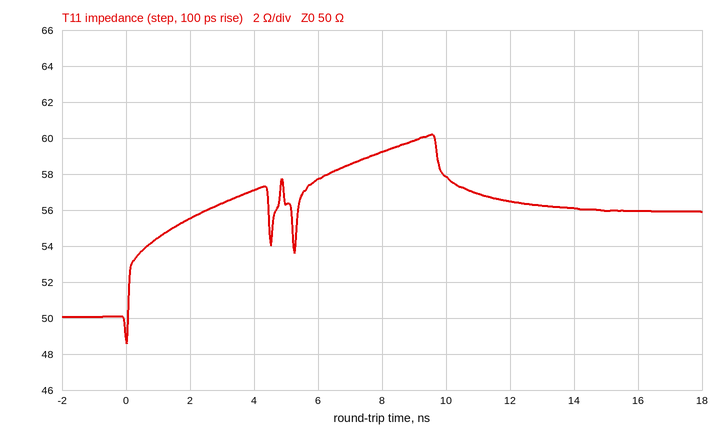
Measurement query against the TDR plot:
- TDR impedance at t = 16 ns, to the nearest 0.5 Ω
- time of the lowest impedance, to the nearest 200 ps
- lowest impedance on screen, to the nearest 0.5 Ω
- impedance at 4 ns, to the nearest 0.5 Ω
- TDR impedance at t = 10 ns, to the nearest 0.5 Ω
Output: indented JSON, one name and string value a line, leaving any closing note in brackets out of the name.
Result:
{
  "TDR impedance at t = 16 ns, to the nearest 0.5 Ω": "56.0 Ω",
  "time of the lowest impedance, to the nearest 200 ps": "0.0 ns",
  "lowest impedance on screen, to the nearest 0.5 Ω": "48.5 Ω",
  "impedance at 4 ns, to the nearest 0.5 Ω": "57.0 Ω",
  "TDR impedance at t = 10 ns, to the nearest 0.5 Ω": "58.0 Ω"
}
